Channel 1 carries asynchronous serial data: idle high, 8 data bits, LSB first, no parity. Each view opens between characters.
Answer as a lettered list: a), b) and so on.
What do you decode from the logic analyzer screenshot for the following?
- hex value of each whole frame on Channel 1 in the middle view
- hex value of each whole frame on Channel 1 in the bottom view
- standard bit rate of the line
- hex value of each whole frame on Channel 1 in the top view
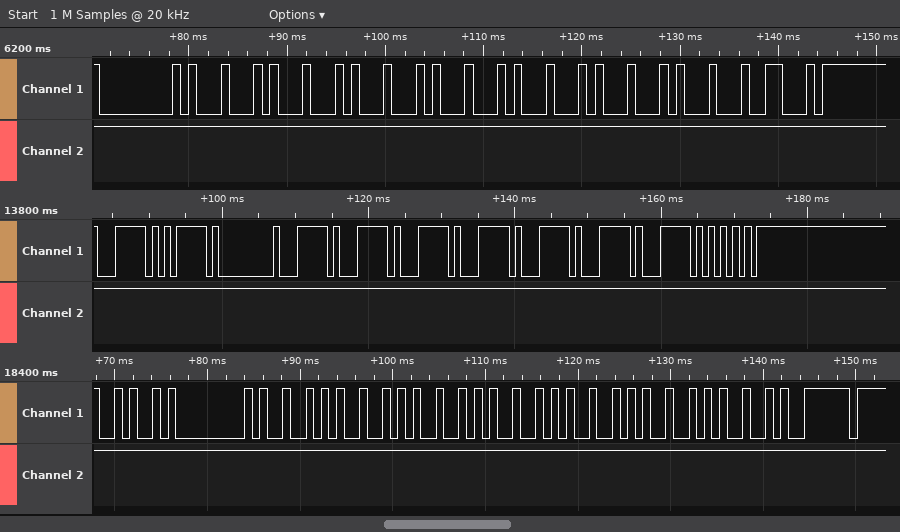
a) 7C, 7D, 00, 7C, 7C, 7C, 7C, 7C, 7C, 7C, 55
b) 4A, 00, 49, 49, 49, 49, 49, 49, 49, 7E
c) 1200 baud
d) 00, 11, 11, 11, 11, 11, 11, 11, 46
